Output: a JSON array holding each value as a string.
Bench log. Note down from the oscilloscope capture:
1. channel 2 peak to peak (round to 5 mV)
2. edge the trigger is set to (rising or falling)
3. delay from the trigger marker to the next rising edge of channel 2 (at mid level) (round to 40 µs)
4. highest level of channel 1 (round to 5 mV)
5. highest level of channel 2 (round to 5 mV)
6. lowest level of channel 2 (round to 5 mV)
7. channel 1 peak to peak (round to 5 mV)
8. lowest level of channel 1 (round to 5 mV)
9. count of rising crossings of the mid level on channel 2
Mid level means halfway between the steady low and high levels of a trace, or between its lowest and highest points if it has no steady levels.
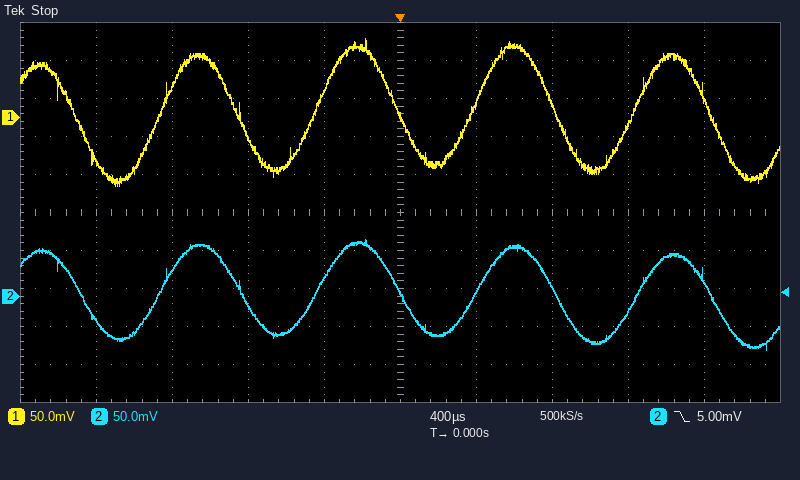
["145 mV", "falling", "400 µs", "105 mV", "75 mV", "-70 mV", "195 mV", "-90 mV", "4"]
